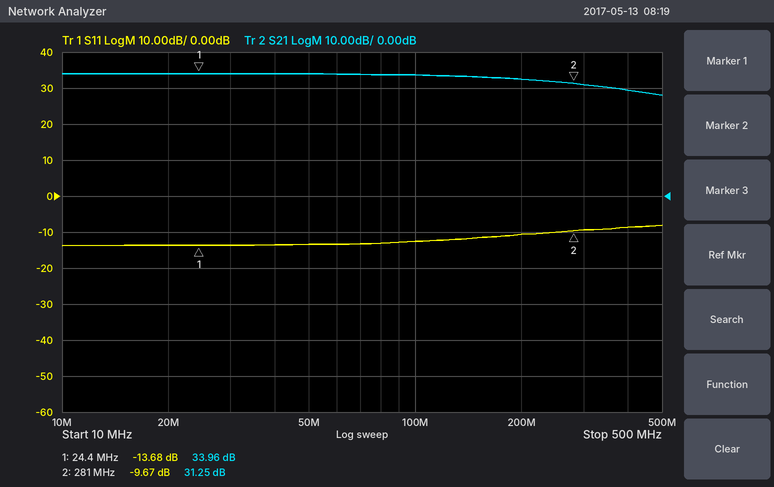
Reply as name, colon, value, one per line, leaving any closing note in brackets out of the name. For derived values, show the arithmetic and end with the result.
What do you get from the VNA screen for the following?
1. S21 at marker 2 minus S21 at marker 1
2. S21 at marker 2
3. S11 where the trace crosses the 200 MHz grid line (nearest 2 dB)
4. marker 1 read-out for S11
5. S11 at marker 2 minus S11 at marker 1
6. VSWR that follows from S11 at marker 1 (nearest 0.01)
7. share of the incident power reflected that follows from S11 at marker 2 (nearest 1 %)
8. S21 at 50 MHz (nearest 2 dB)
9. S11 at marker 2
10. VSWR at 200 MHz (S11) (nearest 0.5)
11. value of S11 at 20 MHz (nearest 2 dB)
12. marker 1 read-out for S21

S21 at marker 2 minus S21 at marker 1: 31.25 − (33.96) = -2.71 dB
S21 at marker 2: 31.25 dB
S11 where the trace crosses the 200 MHz grid line: -10 dB
marker 1 read-out for S11: -13.68 dB
S11 at marker 2 minus S11 at marker 1: -9.67 − (-13.68) = 4.01 dB
VSWR that follows from S11 at marker 1: (1 + 0.2070)/(1 − 0.2070) ≈ 1.52
share of the incident power reflected that follows from S11 at marker 2: 10^(-9.67/10) ≈ 11 %
S21 at 50 MHz: 34 dB
S11 at marker 2: -9.67 dB
VSWR at 200 MHz (S11): |Γ| = 10^(-10/20) = 0.3162; VSWR = (1 + 0.3162)/(1 − 0.3162) ≈ 1.92, so 2.0 to the nearest 0.5
value of S11 at 20 MHz: -14 dB
marker 1 read-out for S21: 33.96 dB
